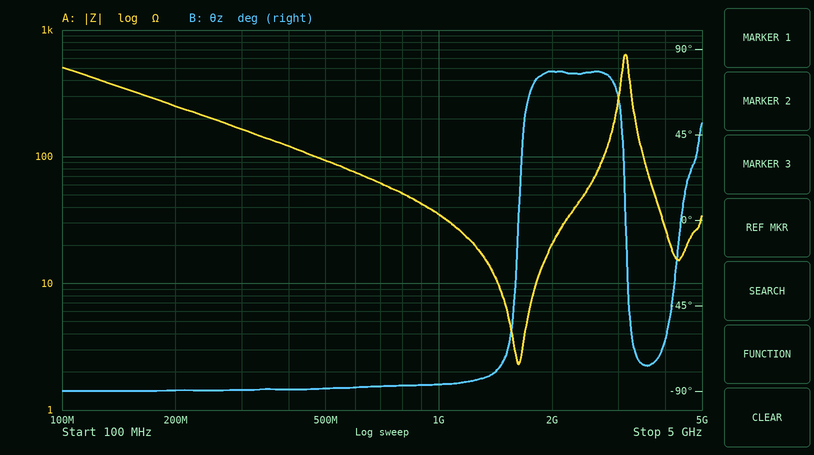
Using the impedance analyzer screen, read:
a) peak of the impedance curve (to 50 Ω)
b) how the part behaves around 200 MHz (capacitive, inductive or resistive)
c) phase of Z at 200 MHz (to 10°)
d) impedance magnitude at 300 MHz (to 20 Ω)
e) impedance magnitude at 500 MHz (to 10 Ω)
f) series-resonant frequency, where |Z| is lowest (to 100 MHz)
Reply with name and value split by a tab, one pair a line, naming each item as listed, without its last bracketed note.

peak of the impedance curve	650 Ω
how the part behaves around 200 MHz	capacitive
phase of Z at 200 MHz	-90°
impedance magnitude at 300 MHz	160 Ω
impedance magnitude at 500 MHz	90 Ω
series-resonant frequency, where |Z| is lowest	1.6 GHz
